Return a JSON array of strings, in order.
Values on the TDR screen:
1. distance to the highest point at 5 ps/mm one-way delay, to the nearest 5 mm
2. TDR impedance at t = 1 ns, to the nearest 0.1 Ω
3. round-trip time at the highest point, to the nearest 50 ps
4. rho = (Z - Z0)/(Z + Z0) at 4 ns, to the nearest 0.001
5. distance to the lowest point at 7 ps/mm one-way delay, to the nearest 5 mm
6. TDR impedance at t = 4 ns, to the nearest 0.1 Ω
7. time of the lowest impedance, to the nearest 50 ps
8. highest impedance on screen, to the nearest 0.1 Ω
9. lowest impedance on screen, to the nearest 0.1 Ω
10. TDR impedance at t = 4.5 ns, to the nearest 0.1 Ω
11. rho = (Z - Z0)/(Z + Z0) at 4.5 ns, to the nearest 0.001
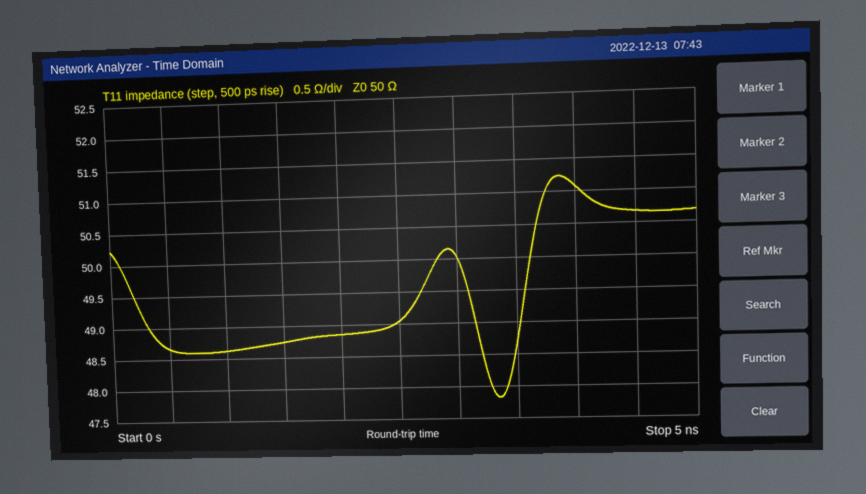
["385 mm", "48.6 Ω", "3.85 ns", "+0.011", "240 mm", "51.1 Ω", "3.35 ns", "51.2 Ω", "47.8 Ω", "50.7 Ω", "+0.007"]
